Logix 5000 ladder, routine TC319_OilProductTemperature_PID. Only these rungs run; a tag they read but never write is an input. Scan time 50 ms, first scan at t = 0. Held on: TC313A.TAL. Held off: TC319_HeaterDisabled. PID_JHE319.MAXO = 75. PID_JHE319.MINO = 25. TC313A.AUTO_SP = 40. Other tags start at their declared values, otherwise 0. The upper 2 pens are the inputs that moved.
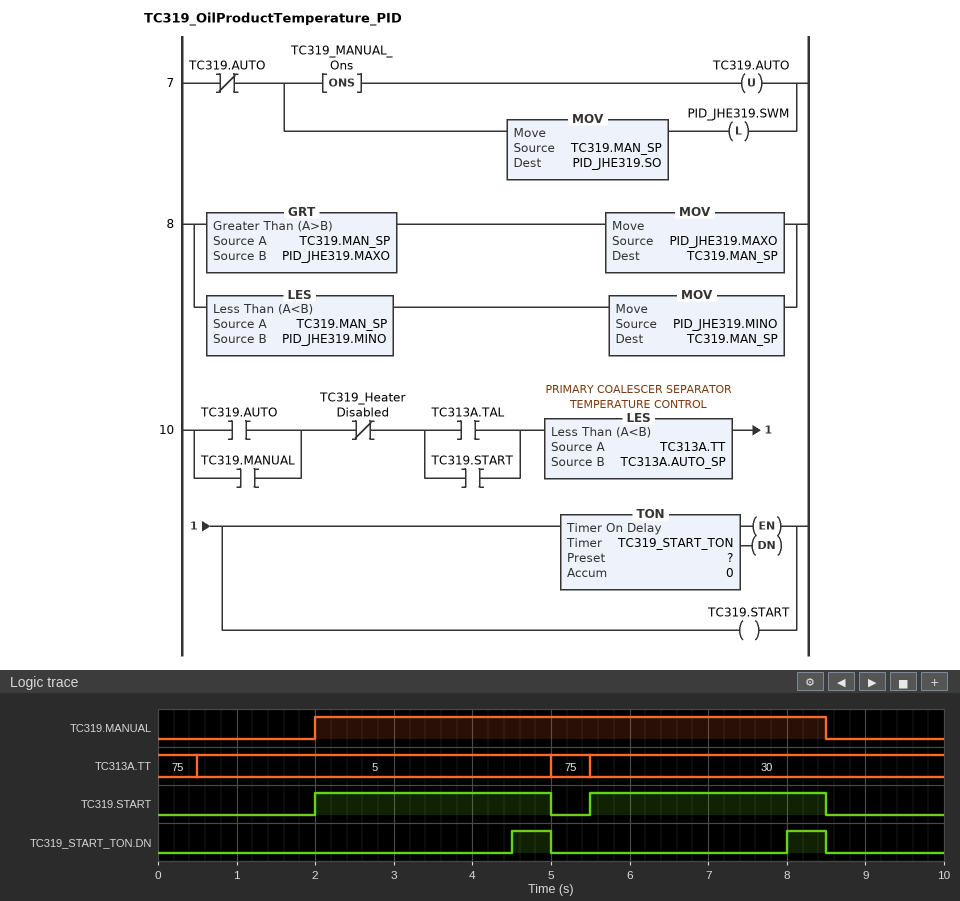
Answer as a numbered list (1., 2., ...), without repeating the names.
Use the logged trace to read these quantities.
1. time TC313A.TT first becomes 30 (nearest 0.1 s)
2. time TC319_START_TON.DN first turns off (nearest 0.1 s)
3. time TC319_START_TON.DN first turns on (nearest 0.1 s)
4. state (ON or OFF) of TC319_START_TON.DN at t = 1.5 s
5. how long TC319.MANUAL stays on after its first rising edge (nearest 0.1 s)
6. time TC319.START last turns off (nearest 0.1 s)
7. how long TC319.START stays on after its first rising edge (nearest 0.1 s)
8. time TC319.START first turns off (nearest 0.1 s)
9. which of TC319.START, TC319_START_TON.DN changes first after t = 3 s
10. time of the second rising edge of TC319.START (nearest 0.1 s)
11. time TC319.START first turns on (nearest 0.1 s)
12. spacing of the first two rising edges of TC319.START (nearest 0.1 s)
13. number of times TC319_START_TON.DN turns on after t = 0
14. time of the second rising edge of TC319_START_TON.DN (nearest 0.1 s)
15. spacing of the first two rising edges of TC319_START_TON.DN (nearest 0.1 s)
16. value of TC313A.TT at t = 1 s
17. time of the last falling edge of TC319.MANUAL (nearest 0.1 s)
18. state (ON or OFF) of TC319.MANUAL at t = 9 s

1. 5.5 s
2. 5.0 s
3. 4.5 s
4. OFF
5. 6.5 s
6. 8.5 s
7. 3.0 s
8. 5.0 s
9. TC319_START_TON.DN
10. 5.5 s
11. 2.0 s
12. 3.5 s
13. 2
14. 8.0 s
15. 3.5 s
16. 5
17. 8.5 s
18. OFF
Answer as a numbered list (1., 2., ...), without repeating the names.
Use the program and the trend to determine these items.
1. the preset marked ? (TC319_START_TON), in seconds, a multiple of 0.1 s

1. 2.5 s
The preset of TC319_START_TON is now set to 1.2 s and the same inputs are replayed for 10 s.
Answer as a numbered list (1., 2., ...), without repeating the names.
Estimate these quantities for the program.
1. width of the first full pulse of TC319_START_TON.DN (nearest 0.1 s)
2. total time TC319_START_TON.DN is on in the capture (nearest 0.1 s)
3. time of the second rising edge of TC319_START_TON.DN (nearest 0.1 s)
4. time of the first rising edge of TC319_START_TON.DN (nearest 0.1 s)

1. 1.8 s
2. 3.6 s
3. 6.7 s
4. 3.2 s
